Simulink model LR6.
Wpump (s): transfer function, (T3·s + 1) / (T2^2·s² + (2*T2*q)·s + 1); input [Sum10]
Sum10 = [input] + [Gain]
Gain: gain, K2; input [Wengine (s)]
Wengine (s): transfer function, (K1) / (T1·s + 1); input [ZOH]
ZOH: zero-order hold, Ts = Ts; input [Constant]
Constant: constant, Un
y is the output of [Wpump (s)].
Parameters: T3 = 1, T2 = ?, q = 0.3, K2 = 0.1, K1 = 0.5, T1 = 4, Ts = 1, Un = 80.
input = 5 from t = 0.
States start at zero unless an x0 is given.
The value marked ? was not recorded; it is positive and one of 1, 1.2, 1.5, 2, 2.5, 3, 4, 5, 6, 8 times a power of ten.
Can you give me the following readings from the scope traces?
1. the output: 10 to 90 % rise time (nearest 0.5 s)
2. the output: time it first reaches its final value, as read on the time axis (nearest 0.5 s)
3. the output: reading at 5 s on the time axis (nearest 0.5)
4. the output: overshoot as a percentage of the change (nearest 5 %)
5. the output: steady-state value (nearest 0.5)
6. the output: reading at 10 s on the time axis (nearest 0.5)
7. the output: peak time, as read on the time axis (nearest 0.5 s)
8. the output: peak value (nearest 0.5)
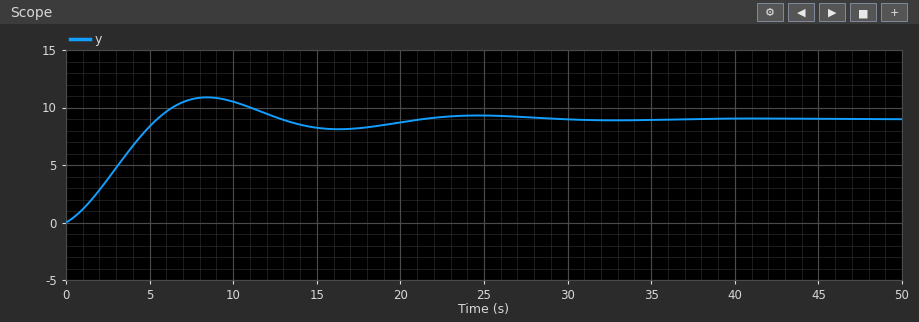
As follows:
4.0 s
5.5 s
8.5
20 %
9.0
10.5
8.5 s
11.0
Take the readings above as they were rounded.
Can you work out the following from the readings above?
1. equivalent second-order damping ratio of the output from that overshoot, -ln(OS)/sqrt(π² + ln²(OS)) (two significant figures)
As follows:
0.46
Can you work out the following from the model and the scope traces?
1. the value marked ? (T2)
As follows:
2.5
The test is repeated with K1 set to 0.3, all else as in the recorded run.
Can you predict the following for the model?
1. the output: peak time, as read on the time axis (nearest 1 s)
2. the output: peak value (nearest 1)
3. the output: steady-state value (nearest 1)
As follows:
8 s
9
7
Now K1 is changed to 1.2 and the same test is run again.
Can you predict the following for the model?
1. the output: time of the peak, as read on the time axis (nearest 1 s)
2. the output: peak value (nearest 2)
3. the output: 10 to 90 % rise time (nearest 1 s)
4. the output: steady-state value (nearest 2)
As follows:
9 s
16
5 s
14
